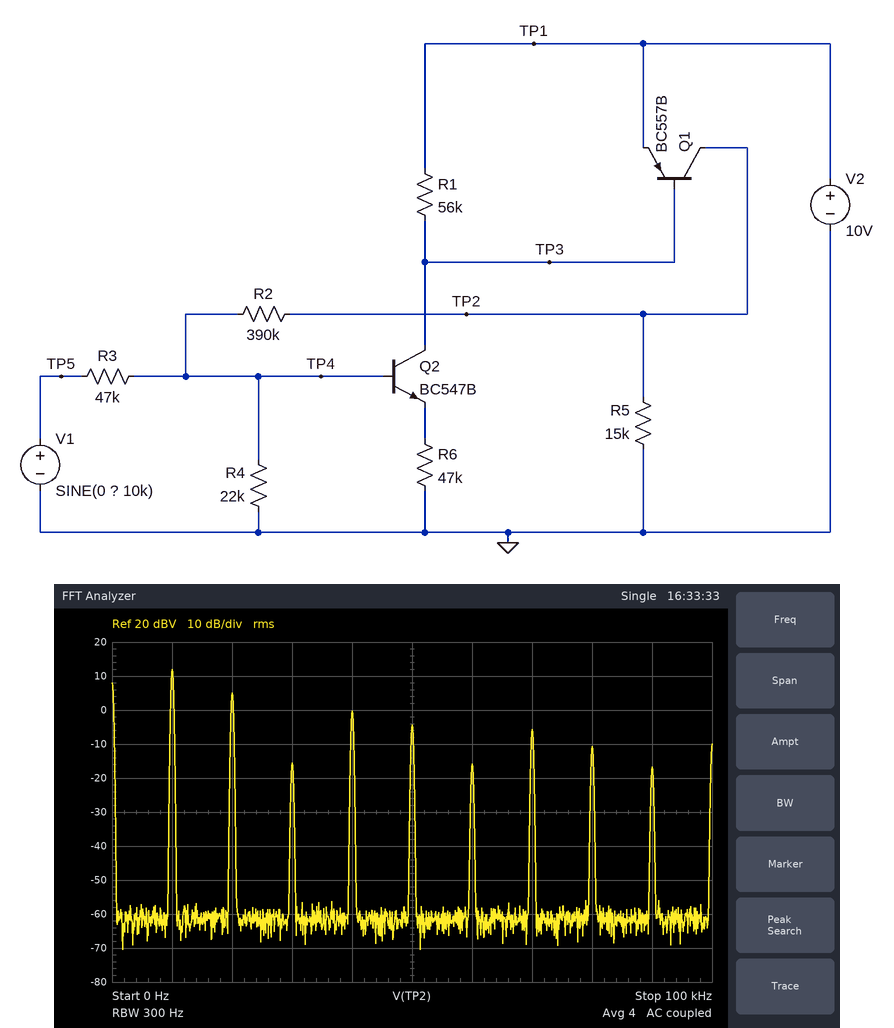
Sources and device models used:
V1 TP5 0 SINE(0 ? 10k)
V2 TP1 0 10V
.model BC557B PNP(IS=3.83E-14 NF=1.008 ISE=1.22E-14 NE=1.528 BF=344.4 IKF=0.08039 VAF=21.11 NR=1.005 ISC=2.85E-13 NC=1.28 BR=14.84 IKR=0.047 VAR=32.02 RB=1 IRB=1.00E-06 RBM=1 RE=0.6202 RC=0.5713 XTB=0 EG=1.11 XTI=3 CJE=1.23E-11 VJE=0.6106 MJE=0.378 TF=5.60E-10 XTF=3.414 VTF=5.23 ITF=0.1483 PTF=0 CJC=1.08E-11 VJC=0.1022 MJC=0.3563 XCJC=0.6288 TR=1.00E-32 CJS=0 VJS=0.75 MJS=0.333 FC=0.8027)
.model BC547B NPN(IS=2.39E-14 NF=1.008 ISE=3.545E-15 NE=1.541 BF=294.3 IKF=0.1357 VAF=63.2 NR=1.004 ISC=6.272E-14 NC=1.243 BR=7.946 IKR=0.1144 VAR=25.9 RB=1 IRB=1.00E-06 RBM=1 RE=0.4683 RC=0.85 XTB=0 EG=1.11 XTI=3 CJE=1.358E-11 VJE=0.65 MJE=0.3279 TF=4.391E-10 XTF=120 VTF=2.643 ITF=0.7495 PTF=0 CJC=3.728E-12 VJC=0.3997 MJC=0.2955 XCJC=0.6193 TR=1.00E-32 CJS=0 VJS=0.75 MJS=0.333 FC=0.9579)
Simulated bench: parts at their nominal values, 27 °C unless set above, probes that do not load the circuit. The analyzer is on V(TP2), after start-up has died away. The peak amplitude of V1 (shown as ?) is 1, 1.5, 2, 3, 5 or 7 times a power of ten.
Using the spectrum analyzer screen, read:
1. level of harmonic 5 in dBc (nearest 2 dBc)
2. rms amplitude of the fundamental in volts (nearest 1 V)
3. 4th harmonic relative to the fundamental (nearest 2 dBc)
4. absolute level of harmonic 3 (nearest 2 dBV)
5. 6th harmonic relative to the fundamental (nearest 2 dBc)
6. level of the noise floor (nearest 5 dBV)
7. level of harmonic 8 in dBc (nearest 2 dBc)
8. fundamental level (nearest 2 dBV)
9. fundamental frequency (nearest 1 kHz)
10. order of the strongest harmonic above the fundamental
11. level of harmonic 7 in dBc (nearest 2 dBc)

-16 dBc
4 V
-12 dBc
-16 dBV
-28 dBc
-60 dBV
-22 dBc
12 dBV
10 kHz
2
-18 dBc
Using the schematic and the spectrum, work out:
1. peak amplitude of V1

5 V
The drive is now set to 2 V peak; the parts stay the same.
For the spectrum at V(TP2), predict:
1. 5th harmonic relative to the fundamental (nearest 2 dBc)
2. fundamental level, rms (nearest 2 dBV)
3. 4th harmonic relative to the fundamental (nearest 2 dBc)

-56 dBc
-36 dBV
-48 dBc
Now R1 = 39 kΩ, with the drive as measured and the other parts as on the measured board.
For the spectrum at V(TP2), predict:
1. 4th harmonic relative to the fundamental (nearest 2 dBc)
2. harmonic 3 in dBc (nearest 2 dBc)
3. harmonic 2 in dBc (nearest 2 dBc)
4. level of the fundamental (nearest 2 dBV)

-18 dBc
-14 dBc
-4 dBc
10 dBV
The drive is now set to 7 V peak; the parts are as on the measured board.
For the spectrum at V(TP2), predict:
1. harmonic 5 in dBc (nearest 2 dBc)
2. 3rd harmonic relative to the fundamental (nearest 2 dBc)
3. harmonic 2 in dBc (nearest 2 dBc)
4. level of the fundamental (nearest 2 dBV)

-40 dBc
-14 dBc
-10 dBc
12 dBV
